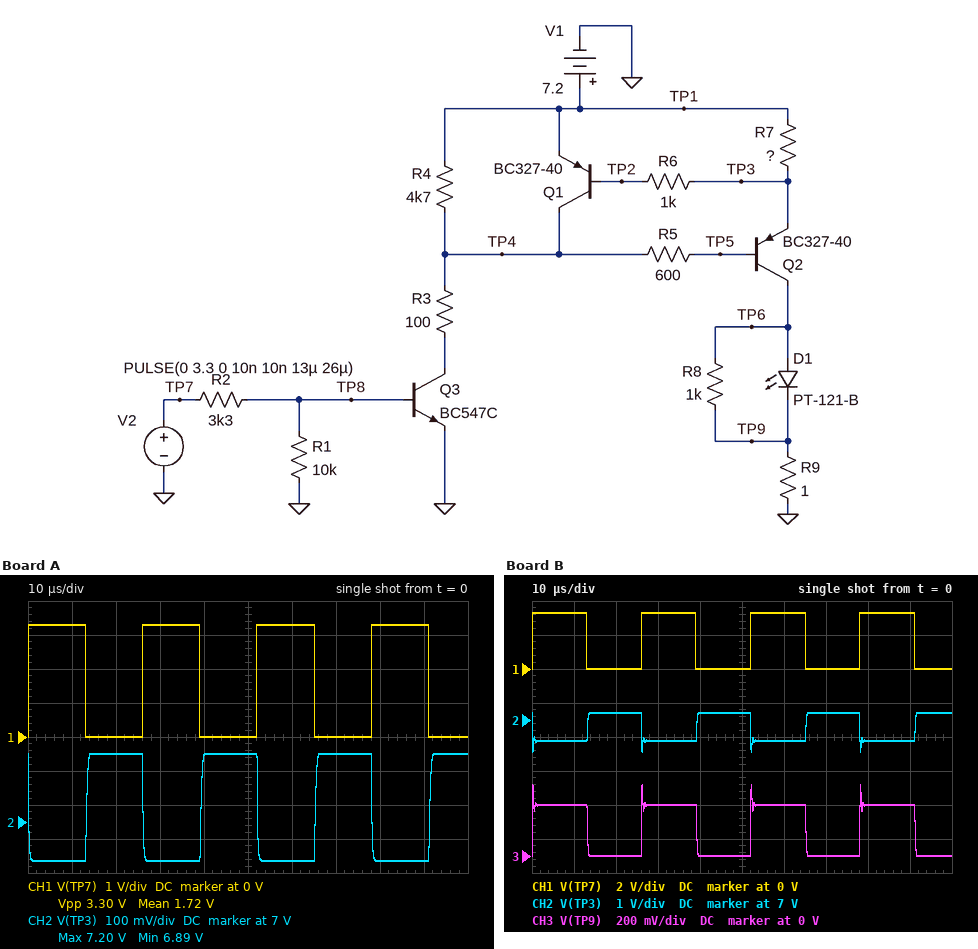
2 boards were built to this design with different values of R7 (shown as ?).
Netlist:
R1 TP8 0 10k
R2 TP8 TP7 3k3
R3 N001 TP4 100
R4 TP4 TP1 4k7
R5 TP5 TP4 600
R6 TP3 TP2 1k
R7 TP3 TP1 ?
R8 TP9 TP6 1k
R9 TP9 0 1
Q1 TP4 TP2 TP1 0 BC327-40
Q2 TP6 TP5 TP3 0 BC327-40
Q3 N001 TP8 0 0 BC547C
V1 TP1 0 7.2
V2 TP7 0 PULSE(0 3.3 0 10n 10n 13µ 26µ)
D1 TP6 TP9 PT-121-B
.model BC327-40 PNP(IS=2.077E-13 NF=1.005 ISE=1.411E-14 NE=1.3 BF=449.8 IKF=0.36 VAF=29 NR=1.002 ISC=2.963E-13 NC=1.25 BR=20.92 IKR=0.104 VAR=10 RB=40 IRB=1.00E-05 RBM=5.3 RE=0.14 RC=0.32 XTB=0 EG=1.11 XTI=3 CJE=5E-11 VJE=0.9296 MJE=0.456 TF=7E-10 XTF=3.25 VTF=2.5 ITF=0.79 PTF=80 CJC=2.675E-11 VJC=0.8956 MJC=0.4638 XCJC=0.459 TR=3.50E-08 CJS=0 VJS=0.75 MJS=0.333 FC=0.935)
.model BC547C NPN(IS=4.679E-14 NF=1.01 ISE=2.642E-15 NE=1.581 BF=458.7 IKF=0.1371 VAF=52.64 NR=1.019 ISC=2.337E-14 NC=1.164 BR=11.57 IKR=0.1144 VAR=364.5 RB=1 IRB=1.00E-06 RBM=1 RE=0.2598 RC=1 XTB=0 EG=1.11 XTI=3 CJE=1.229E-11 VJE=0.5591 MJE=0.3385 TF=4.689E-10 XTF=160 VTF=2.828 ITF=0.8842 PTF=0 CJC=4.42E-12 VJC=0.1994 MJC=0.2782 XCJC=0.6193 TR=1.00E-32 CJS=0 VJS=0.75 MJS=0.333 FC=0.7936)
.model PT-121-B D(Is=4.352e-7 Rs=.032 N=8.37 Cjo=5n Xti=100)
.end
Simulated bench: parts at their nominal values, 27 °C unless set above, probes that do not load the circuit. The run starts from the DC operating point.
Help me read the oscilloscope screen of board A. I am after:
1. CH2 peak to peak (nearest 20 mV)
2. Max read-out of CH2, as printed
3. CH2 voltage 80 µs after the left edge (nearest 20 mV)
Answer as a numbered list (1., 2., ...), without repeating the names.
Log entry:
1. 320 mV
2. 7.20 V
3. 6.88 V
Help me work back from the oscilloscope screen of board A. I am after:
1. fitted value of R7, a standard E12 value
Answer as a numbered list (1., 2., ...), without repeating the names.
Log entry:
1. 0.33 Ω
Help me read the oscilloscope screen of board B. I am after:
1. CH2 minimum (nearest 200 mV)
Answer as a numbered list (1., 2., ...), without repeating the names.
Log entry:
1. 6.0 V
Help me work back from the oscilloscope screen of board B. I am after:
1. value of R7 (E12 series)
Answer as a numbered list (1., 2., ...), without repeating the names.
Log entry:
1. 2.7 Ω
